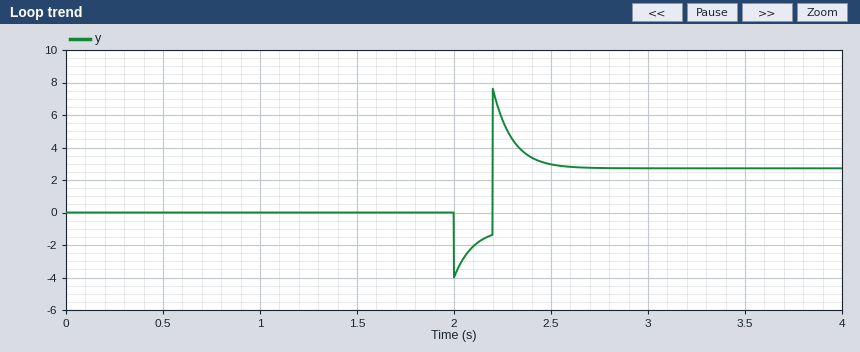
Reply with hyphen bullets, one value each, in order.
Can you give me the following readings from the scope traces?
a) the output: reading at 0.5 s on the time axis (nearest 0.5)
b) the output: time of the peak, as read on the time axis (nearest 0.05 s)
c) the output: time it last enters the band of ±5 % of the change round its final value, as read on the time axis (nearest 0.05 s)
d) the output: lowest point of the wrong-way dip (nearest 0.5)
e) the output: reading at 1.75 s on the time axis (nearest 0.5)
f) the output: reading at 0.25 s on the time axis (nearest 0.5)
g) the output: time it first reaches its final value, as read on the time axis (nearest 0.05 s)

- 0.0
- 2.20 s
- 2.55 s
- -4.0
- 0.0
- 0.0
- 2.20 s
